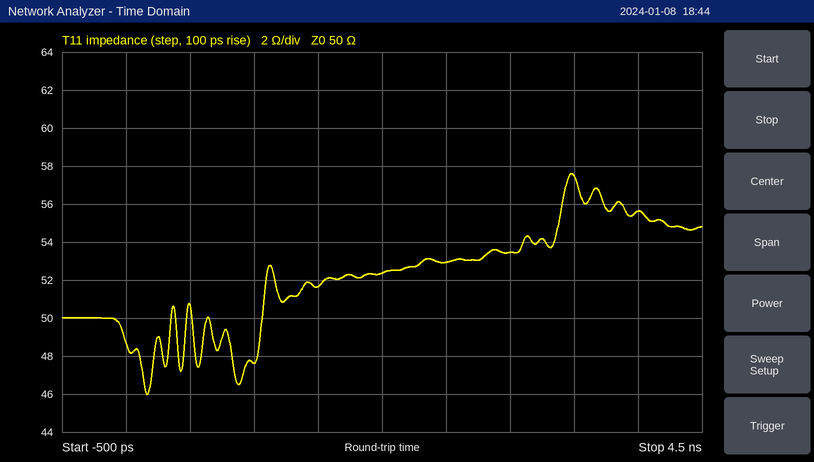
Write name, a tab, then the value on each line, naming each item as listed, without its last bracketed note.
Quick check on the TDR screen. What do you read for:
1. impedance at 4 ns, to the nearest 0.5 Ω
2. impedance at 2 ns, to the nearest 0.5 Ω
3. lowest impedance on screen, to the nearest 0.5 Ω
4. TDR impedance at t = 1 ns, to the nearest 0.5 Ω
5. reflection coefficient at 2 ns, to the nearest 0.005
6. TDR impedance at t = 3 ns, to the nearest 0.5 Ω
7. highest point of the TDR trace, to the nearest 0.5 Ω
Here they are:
impedance at 4 ns, to the nearest 0.5 Ω	55.5 Ω
impedance at 2 ns, to the nearest 0.5 Ω	52.5 Ω
lowest impedance on screen, to the nearest 0.5 Ω	46.0 Ω
TDR impedance at t = 1 ns, to the nearest 0.5 Ω	47.5 Ω
reflection coefficient at 2 ns, to the nearest 0.005	+0.025
TDR impedance at t = 3 ns, to the nearest 0.5 Ω	53.5 Ω
highest point of the TDR trace, to the nearest 0.5 Ω	57.5 Ω
